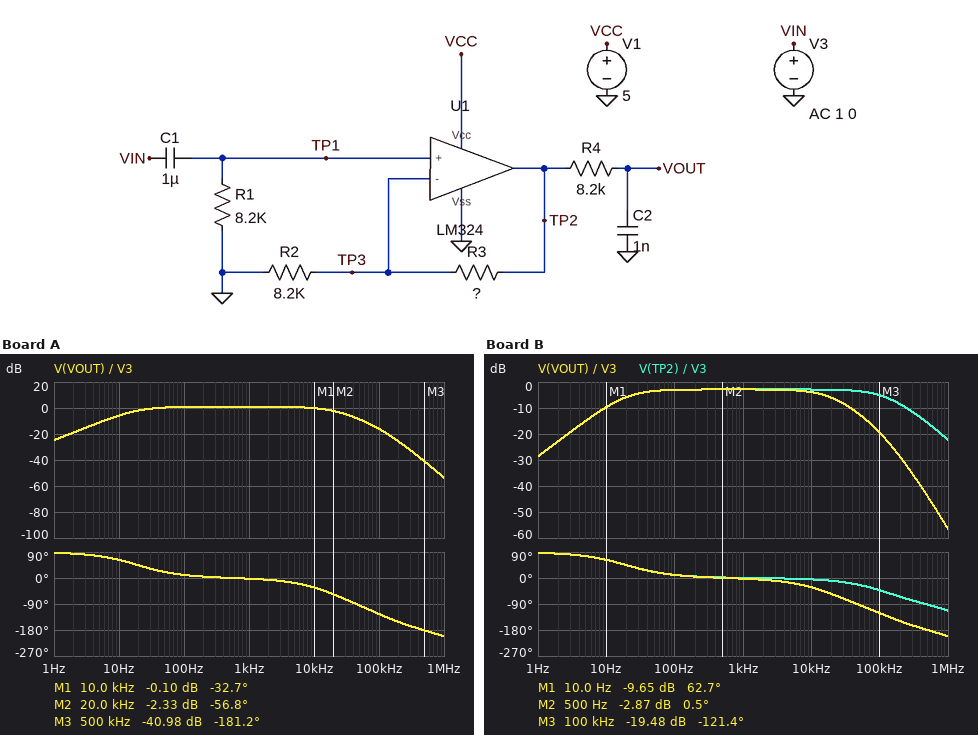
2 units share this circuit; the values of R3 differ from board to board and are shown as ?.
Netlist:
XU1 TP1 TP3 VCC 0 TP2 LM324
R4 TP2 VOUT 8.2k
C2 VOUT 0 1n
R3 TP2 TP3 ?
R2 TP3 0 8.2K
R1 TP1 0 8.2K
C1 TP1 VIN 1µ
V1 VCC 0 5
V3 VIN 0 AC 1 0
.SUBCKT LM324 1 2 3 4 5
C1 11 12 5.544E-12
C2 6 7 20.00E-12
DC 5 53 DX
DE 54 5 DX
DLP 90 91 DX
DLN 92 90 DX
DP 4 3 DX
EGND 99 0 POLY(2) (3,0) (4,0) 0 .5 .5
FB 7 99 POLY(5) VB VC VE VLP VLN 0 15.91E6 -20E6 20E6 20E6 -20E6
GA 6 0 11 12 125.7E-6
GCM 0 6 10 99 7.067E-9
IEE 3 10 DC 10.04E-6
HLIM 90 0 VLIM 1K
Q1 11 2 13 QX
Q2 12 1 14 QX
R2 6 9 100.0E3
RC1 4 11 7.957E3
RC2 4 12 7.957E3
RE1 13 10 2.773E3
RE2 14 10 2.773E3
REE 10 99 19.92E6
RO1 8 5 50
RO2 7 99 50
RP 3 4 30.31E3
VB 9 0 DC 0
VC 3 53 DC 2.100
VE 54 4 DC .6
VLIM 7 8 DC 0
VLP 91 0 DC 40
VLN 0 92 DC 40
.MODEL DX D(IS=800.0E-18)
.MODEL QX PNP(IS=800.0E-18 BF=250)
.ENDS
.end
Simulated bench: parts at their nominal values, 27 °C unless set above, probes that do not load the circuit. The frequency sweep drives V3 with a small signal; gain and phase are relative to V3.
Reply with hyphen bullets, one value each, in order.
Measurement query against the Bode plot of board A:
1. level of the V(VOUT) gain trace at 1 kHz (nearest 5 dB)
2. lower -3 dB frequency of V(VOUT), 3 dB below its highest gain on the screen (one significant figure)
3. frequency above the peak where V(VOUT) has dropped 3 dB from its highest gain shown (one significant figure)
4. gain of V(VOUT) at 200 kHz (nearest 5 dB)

- 0 dB
- 20 Hz
- 20 kHz
- -25 dB
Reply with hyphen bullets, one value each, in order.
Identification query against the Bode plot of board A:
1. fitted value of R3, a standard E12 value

- 18 kΩ
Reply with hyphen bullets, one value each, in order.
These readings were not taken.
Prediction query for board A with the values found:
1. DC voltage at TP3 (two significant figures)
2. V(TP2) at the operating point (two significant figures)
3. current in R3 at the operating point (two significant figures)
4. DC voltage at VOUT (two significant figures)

- 15 mV
- 48 mV
- 1.8 µA
- 48 mV
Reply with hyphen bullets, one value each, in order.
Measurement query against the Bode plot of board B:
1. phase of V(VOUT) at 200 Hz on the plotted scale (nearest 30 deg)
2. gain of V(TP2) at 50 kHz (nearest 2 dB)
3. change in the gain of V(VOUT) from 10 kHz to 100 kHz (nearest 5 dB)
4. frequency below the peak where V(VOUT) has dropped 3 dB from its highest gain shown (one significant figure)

- 0 deg
- -4 dB
- -15 dB
- 20 Hz
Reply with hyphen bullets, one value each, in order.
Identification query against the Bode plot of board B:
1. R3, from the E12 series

- 6.8 kΩ
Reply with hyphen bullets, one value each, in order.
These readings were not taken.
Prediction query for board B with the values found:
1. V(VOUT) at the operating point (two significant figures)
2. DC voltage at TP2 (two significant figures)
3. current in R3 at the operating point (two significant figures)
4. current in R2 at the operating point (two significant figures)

- 39 mV
- 39 mV
- 2.6 µA
- 2.6 µA
